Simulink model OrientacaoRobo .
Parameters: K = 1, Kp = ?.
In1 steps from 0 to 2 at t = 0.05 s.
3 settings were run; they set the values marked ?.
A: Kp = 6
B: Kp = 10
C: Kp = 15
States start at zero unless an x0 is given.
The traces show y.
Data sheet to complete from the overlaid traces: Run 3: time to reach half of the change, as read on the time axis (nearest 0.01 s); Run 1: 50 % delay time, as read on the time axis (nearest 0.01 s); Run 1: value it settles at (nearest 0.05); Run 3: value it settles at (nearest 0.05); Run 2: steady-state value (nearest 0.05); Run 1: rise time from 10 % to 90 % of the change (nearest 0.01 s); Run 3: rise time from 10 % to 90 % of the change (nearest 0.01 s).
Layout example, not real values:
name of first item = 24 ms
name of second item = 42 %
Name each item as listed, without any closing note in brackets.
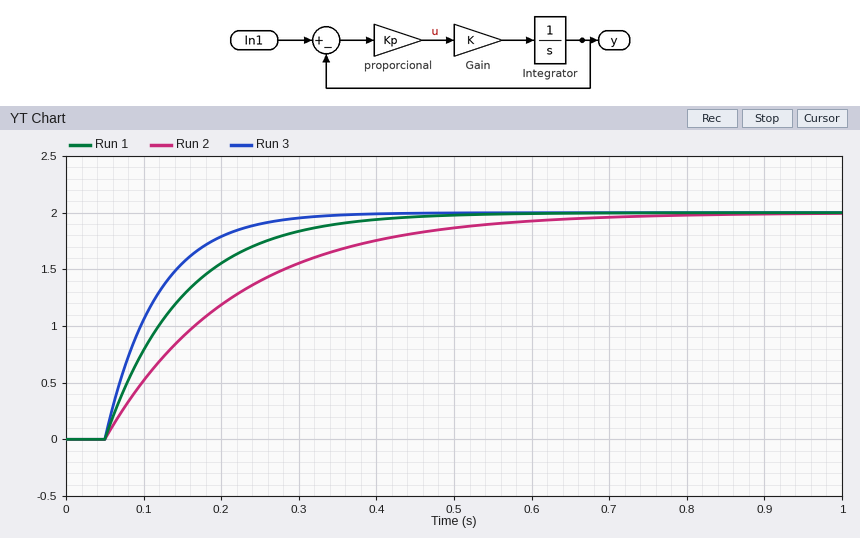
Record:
Run 3: time to reach half of the change, as read on the time axis = 0.10 s
Run 1: 50 % delay time, as read on the time axis = 0.12 s
Run 1: value it settles at = 2.00
Run 3: value it settles at = 2.00
Run 2: steady-state value = 2.00
Run 1: rise time from 10 % to 90 % of the change = 0.22 s
Run 3: rise time from 10 % to 90 % of the change = 0.15 s
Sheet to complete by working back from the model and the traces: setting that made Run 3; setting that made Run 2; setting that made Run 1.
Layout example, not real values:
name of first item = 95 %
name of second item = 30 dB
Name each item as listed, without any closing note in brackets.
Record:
setting that made Run 3 = C
setting that made Run 2 = A
setting that made Run 1 = B
